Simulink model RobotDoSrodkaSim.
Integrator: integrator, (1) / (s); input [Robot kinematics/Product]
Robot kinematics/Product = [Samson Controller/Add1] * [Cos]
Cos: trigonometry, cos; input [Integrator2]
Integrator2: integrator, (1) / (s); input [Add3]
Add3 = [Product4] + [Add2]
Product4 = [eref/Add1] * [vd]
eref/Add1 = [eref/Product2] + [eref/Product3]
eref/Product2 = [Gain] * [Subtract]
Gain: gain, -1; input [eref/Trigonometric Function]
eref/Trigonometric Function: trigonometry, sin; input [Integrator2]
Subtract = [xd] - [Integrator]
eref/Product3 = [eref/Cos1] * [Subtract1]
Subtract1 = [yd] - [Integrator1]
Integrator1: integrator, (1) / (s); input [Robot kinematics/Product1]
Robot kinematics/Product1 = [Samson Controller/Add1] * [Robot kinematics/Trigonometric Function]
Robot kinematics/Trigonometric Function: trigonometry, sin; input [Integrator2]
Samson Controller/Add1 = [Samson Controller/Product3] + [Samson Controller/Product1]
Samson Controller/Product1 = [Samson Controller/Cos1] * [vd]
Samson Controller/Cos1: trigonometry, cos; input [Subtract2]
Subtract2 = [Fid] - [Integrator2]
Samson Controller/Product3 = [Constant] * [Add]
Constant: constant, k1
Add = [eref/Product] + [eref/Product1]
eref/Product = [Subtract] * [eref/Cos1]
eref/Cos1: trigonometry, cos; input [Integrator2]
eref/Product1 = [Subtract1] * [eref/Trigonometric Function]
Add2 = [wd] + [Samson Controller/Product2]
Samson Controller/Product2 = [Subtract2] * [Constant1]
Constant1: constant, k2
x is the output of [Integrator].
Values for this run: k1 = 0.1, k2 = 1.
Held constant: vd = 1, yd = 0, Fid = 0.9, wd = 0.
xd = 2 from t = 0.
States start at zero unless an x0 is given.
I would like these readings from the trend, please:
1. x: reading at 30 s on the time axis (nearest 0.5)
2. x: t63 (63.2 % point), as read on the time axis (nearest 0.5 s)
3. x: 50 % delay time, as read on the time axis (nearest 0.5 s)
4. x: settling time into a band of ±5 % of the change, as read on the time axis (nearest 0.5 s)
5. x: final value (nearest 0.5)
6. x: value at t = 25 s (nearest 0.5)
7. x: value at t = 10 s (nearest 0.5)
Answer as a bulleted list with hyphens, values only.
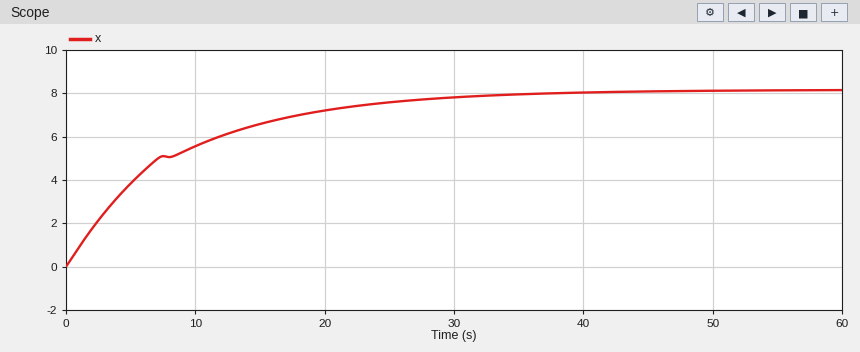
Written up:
- 8.0
- 8.5 s
- 5.5 s
- 28.5 s
- 8.0
- 7.5
- 5.5
